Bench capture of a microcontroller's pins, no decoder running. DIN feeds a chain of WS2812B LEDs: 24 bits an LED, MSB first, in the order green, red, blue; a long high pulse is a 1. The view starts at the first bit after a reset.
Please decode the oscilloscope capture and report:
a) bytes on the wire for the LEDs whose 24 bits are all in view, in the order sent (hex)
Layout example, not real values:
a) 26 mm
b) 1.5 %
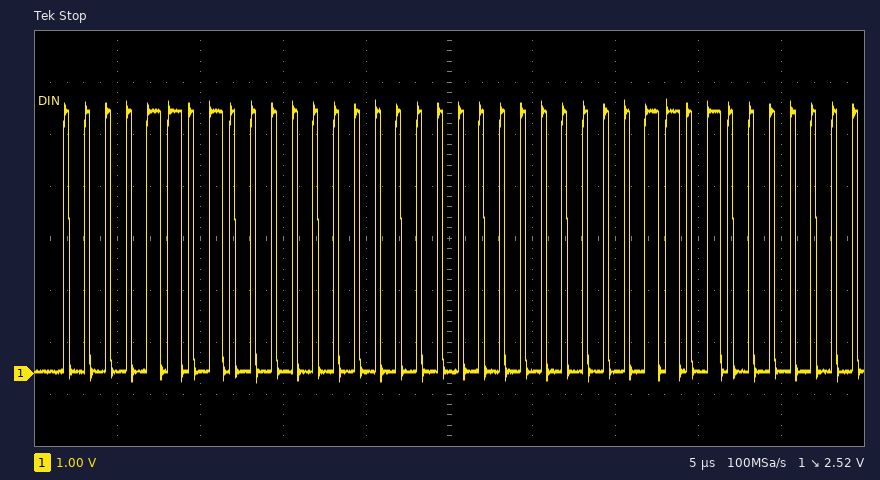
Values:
a) 0D 00 00
